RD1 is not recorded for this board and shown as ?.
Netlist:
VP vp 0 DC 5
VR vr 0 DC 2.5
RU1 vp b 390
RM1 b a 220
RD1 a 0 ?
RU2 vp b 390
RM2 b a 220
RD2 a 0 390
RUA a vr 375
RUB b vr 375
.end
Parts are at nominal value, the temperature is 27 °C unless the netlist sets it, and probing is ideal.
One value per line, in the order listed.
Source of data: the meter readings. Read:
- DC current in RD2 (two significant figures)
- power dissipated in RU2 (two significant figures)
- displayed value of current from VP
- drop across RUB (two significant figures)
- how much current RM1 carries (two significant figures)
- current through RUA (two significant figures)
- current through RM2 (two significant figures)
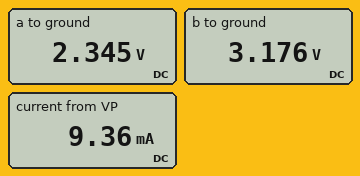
6.0 mA
8.5 mW
9.36 mA
680 mV
3.8 mA
410 µA
3.8 mA
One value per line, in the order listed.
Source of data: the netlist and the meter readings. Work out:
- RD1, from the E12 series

1.2 kΩ
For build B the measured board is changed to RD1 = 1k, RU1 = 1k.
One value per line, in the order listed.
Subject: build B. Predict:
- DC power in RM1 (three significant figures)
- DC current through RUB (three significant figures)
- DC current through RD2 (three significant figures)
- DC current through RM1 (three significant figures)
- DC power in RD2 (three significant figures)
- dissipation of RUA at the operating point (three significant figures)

2.42 mW
973 µA
5.47 mA
3.32 mA
11.7 mW
355 µW
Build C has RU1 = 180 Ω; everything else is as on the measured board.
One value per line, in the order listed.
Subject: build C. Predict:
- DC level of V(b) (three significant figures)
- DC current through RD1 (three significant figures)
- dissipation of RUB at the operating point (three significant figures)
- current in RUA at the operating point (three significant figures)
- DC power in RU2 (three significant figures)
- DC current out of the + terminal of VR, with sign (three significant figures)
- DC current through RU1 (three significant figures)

3.55 V
2.14 mA
2.96 mW
192 µA
5.36 mW
-3.00 mA
8.03 mA
